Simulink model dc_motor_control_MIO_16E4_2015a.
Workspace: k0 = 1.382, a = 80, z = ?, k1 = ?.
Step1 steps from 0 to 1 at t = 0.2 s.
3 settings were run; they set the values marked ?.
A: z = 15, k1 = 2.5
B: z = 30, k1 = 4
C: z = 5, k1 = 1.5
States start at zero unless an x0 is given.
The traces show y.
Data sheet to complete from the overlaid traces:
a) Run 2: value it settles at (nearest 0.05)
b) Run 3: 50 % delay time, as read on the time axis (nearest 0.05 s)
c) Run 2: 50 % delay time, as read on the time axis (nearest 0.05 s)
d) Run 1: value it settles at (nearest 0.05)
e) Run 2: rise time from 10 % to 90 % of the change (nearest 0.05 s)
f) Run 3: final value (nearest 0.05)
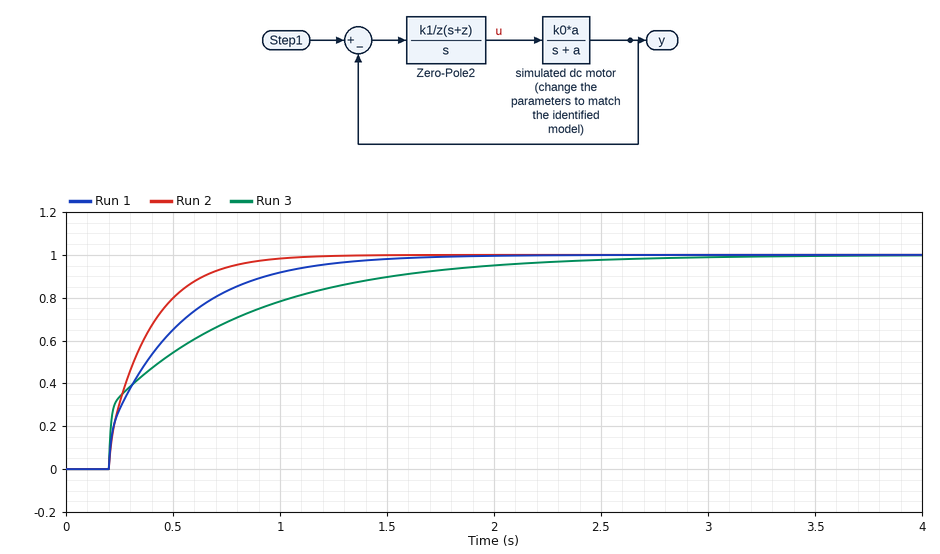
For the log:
1.00
0.45 s
0.30 s
1.00
0.45 s
1.00
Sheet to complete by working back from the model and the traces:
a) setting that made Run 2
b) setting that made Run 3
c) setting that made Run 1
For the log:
B
C
A
